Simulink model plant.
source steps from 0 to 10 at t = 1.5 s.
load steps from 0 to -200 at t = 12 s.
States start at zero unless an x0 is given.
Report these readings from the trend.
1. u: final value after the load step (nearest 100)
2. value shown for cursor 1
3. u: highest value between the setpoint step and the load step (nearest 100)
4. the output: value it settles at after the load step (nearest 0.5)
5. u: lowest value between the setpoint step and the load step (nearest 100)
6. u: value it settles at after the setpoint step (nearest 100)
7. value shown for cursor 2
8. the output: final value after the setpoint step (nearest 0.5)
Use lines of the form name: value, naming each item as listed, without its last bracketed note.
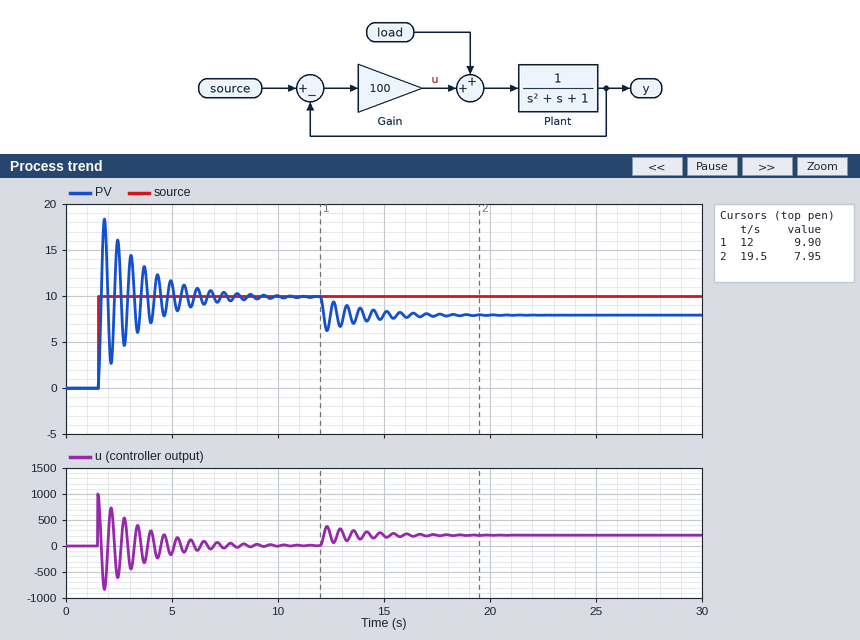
u: final value after the load step: 200
value shown for cursor 1: 9.90
u: highest value between the setpoint step and the load step: 1000
the output: value it settles at after the load step: 8.0
u: lowest value between the setpoint step and the load step: -800
u: value it settles at after the setpoint step: 0
value shown for cursor 2: 7.95
the output: final value after the setpoint step: 10.0
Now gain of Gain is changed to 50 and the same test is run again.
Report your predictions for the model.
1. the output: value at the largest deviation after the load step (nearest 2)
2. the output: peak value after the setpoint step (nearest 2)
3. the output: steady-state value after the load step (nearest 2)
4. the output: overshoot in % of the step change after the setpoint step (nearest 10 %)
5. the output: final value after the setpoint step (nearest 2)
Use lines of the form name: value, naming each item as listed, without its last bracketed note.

the output: value at the largest deviation after the load step: 2
the output: peak value after the setpoint step: 18
the output: steady-state value after the load step: 6
the output: overshoot in % of the step change after the setpoint step: 80 %
the output: final value after the setpoint step: 10
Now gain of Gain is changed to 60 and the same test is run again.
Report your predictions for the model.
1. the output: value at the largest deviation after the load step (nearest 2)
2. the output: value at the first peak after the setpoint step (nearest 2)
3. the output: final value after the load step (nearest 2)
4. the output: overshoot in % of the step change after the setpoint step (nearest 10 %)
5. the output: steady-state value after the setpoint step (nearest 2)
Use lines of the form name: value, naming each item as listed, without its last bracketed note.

the output: value at the largest deviation after the load step: 4
the output: value at the first peak after the setpoint step: 18
the output: final value after the load step: 6
the output: overshoot in % of the step change after the setpoint step: 80 %
the output: steady-state value after the setpoint step: 10
